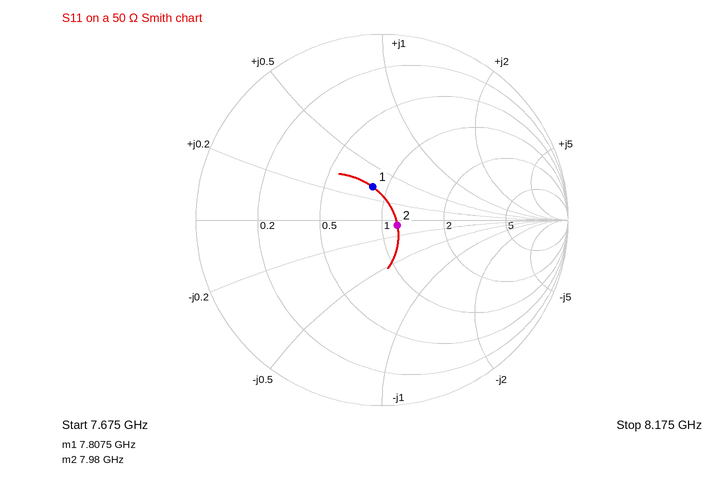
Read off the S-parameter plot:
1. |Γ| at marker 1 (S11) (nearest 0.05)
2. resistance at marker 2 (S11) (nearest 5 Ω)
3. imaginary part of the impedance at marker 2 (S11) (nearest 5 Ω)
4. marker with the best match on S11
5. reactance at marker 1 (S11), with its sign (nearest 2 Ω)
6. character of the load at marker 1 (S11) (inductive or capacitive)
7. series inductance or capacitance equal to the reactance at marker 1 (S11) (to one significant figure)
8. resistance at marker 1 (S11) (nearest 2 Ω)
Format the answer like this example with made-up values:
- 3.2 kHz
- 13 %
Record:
- 0.20
- 60 Ω
- -5 Ω
- marker 2
- +16 Ω
- inductive
- 300 pH
- 42 Ω
